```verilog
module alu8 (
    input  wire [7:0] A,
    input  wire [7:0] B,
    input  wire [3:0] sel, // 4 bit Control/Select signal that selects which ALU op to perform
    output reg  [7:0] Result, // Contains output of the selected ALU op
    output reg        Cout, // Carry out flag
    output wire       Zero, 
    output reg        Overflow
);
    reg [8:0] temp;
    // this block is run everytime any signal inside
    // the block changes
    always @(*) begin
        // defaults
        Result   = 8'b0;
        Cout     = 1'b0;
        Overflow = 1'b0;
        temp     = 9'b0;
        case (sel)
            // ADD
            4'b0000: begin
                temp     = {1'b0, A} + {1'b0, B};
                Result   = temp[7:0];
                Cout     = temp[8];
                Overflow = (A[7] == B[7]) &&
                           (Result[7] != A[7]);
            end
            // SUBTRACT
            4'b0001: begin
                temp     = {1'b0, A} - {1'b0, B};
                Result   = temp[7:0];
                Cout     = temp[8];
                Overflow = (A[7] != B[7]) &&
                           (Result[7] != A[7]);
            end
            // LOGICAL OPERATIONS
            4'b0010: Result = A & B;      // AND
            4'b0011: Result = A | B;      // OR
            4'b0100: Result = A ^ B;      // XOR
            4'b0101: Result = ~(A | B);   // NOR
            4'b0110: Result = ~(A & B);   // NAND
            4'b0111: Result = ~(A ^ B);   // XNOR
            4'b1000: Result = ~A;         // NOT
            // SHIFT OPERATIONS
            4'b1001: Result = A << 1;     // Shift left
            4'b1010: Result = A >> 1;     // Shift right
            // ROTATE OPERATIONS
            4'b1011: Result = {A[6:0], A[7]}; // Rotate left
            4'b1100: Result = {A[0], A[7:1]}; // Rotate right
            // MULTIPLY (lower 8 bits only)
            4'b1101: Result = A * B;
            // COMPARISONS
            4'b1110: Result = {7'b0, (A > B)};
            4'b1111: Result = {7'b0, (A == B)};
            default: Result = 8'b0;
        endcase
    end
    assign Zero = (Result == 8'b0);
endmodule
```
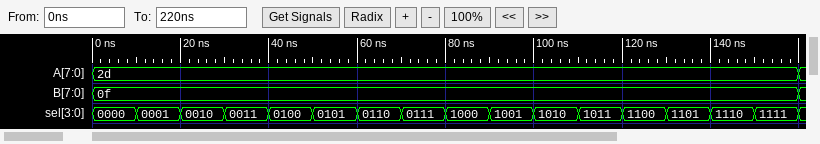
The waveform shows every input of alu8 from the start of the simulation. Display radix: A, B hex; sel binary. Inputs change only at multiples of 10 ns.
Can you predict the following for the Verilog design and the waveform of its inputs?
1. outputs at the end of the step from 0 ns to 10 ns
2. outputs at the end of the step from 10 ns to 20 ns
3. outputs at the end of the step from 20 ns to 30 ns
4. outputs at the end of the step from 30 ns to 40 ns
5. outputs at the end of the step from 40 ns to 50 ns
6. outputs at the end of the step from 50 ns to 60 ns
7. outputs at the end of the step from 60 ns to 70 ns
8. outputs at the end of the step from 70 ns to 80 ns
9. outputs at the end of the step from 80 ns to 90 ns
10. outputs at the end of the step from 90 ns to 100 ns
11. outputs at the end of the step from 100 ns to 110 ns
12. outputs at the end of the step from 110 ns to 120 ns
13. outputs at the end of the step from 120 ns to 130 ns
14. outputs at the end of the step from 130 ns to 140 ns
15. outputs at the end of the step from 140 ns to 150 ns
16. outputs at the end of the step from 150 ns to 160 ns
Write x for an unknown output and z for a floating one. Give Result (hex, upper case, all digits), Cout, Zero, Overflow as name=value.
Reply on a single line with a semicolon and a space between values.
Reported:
Result=3C, Cout=0, Zero=0, Overflow=0; Result=1E, Cout=0, Zero=0, Overflow=0; Result=0D, Cout=0, Zero=0, Overflow=0; Result=2F, Cout=0, Zero=0, Overflow=0; Result=22, Cout=0, Zero=0, Overflow=0; Result=D0, Cout=0, Zero=0, Overflow=0; Result=F2, Cout=0, Zero=0, Overflow=0; Result=DD, Cout=0, Zero=0, Overflow=0; Result=D2, Cout=0, Zero=0, Overflow=0; Result=5A, Cout=0, Zero=0, Overflow=0; Result=16, Cout=0, Zero=0, Overflow=0; Result=5A, Cout=0, Zero=0, Overflow=0; Result=96, Cout=0, Zero=0, Overflow=0; Result=A3, Cout=0, Zero=0, Overflow=0; Result=01, Cout=0, Zero=0, Overflow=0; Result=00, Cout=0, Zero=1, Overflow=0
